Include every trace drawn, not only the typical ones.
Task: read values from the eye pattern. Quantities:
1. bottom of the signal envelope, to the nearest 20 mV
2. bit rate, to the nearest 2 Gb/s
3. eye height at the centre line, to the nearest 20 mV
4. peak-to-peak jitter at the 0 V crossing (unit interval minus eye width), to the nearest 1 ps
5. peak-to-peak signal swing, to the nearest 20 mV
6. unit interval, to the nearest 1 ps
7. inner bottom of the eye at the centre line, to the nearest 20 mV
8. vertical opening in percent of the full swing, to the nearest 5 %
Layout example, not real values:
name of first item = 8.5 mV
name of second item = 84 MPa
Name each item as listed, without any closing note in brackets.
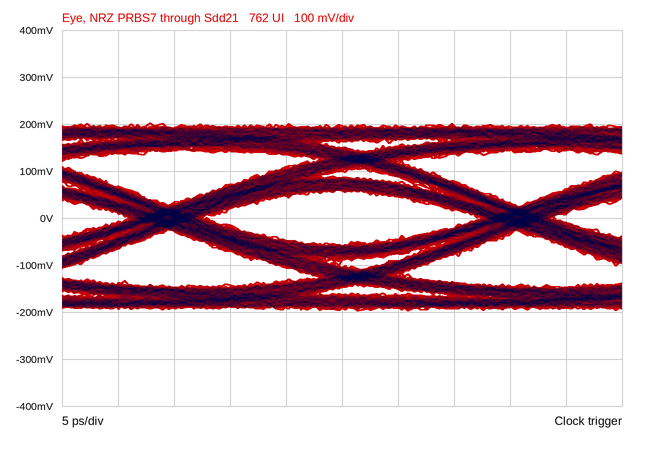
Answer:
bottom of the signal envelope, to the nearest 20 mV = -200 mV
bit rate, to the nearest 2 Gb/s = 32 Gb/s
eye height at the centre line, to the nearest 20 mV = 120 mV
peak-to-peak jitter at the 0 V crossing (unit interval minus eye width), to the nearest 1 ps = 7 ps
peak-to-peak signal swing, to the nearest 20 mV = 400 mV
unit interval, to the nearest 1 ps = 31 ps
inner bottom of the eye at the centre line, to the nearest 20 mV = -60 mV
vertical opening in percent of the full swing, to the nearest 5 % = 30 %
